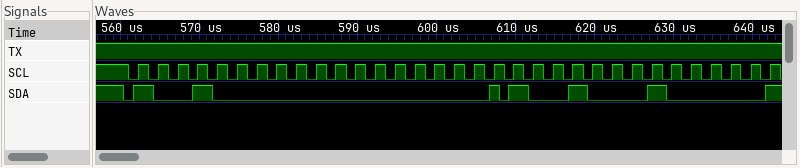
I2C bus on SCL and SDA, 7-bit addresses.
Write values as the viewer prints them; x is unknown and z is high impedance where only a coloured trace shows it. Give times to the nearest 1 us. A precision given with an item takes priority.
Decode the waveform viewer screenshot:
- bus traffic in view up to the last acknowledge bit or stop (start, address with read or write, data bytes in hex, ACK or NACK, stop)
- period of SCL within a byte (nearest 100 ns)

start, address 48 write ACK, 00 ACK, repeated start, address 48 read ACK
2500 ns
